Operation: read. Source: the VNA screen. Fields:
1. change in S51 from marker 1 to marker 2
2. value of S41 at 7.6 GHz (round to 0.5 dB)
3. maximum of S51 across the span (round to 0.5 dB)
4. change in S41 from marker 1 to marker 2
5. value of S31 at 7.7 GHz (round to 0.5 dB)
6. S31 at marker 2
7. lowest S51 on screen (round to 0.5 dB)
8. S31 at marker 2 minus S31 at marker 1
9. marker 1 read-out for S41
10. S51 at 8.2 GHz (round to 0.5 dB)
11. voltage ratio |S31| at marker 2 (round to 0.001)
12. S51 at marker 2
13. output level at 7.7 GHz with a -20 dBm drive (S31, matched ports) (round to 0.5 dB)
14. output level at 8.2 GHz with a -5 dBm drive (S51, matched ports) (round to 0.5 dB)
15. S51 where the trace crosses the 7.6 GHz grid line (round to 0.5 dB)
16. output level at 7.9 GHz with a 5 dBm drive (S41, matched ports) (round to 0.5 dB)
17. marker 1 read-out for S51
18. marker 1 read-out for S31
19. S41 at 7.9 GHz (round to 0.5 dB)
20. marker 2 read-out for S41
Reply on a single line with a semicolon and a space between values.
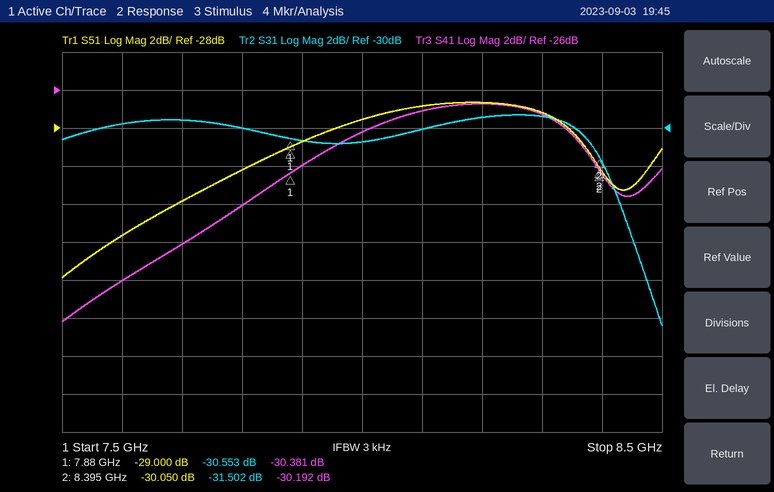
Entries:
-1.050 dB; -36.0 dB; -26.5 dB; 0.189 dB; -29.5 dB; -31.502 dB; -36.0 dB; -0.949 dB; -30.381 dB; -26.5 dB; 0.027; -30.050 dB; -49.5 dBm; -31.5 dBm; -33.5 dB; -25.0 dBm; -29.000 dB; -30.553 dB; -30.0 dB; -30.192 dB
